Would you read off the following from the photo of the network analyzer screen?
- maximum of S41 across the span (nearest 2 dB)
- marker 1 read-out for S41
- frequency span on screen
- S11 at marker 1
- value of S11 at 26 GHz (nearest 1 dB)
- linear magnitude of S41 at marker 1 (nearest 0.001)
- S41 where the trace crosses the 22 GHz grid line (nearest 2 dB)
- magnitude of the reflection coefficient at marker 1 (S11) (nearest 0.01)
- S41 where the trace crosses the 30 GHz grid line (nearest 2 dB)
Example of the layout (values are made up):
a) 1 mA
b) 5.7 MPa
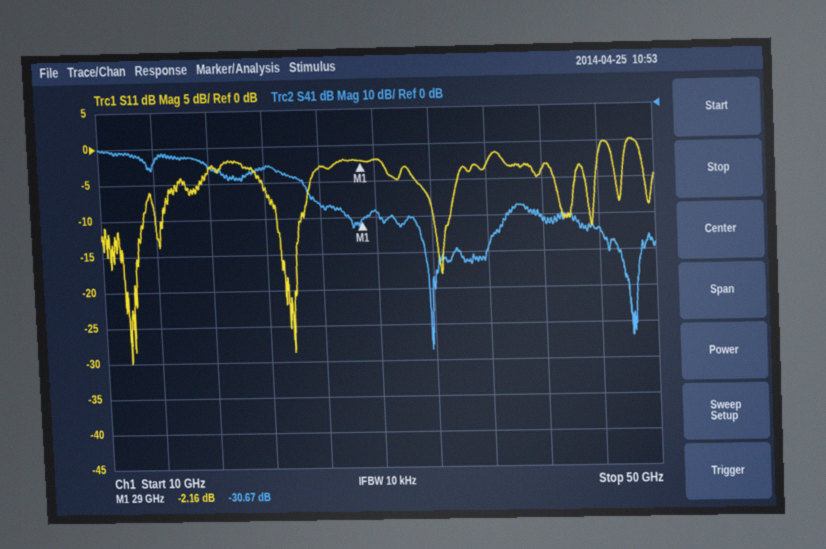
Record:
a) -10 dB
b) -30.67 dB
c) 40 GHz
d) -2.16 dB
e) -3 dB
f) 0.029
g) -16 dB
h) 0.78
i) -28 dB
